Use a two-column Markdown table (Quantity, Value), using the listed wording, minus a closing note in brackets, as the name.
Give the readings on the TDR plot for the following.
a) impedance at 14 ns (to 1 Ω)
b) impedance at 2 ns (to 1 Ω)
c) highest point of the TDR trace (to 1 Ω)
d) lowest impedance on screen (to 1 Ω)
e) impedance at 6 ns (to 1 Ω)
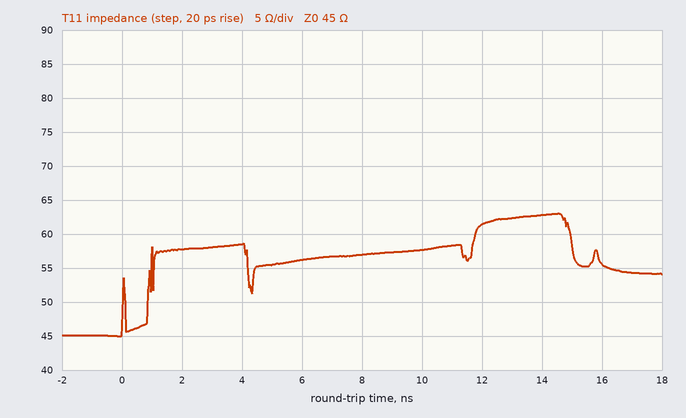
| Quantity | Value |
|---|---|
| impedance at 14 ns | 63 Ω |
| impedance at 2 ns | 58 Ω |
| highest point of the TDR trace | 63 Ω |
| lowest impedance on screen | 45 Ω |
| impedance at 6 ns | 56 Ω |
